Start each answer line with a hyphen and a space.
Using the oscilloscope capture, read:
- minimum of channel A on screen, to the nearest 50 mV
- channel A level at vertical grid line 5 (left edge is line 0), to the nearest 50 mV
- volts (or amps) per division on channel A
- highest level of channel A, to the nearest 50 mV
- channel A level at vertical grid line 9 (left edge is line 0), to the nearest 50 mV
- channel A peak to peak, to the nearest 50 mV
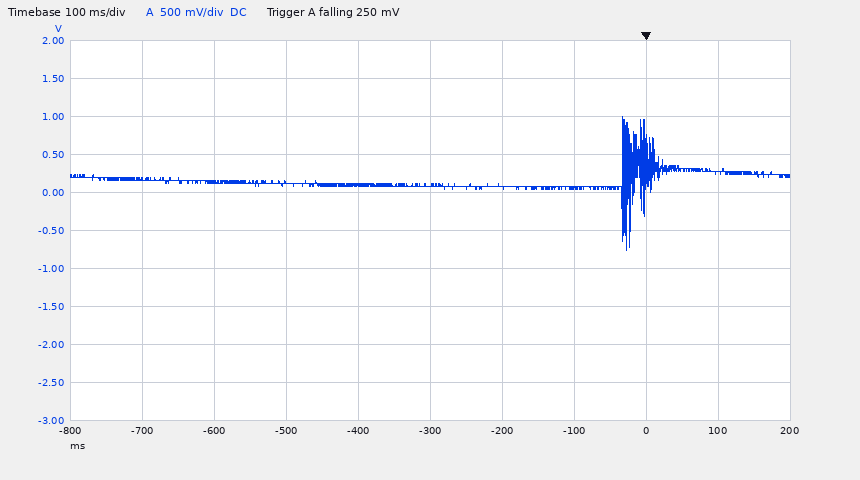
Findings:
- -750 mV
- 100 mV
- 500 mV
- 1.00 V
- 250 mV
- 1.75 V
